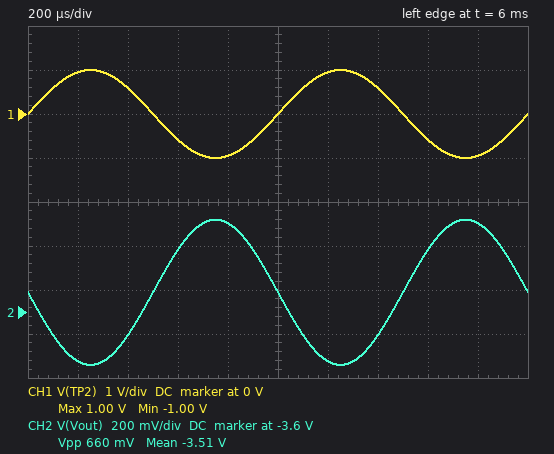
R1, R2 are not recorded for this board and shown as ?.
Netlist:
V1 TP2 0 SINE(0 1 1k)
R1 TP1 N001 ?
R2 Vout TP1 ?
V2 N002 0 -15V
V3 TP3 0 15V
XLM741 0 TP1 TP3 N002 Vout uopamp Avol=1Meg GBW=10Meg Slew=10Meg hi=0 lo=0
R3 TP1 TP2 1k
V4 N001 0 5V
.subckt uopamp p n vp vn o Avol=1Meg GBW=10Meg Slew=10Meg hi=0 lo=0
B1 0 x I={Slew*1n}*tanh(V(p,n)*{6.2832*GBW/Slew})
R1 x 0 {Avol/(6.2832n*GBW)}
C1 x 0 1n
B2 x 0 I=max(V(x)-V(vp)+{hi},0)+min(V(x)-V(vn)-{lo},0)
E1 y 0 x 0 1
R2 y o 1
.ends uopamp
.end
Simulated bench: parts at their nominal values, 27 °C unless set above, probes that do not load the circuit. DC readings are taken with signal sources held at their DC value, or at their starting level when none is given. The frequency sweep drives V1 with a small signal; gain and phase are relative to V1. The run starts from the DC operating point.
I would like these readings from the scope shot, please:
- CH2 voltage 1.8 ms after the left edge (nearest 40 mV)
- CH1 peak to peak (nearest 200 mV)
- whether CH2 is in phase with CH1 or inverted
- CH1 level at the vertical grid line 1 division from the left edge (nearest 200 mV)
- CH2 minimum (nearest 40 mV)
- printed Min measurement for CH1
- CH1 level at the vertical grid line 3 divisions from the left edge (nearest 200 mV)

-3.20 V
2.0 V
inverted
1.0 V
-3.84 V
-1.00 V
-600 mV
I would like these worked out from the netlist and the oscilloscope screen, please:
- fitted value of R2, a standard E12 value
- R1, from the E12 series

330 Ω
470 Ω
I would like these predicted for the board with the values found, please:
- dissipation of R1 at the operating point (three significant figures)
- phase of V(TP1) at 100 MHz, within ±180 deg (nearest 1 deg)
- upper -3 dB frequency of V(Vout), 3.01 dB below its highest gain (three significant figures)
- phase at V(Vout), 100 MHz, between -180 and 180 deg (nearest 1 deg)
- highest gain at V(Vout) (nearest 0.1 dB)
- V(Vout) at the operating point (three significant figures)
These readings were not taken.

53.2 mW
3 deg
4.91 MHz
91 deg
-9.6 dB
-3.51 V
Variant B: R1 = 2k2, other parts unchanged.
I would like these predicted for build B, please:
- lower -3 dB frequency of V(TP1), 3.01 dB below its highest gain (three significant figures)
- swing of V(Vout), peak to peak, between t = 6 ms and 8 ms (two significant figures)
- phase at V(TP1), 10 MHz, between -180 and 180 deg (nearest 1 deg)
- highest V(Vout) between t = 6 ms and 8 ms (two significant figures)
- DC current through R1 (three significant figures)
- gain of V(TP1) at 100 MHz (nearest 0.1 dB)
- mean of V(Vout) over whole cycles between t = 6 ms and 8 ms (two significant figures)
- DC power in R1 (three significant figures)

6.75 MHz
660 mV
34 deg
-420 mV
2.27 mA
-13.0 dB
-750 mV
11.4 mW
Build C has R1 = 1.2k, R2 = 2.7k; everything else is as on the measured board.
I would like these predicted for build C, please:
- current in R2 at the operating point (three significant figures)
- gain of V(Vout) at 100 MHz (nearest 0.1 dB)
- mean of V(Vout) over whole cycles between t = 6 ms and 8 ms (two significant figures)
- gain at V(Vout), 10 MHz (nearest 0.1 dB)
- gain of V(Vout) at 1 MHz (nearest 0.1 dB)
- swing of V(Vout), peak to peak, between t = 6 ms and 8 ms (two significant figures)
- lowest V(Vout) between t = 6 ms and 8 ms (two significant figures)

4.17 mA
-26.9 dB
-11 V
-7.0 dB
7.3 dB
5.4 V
-14 V
